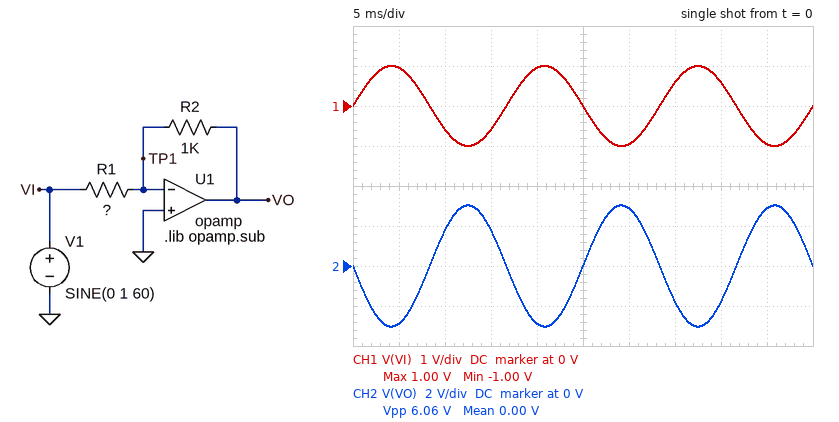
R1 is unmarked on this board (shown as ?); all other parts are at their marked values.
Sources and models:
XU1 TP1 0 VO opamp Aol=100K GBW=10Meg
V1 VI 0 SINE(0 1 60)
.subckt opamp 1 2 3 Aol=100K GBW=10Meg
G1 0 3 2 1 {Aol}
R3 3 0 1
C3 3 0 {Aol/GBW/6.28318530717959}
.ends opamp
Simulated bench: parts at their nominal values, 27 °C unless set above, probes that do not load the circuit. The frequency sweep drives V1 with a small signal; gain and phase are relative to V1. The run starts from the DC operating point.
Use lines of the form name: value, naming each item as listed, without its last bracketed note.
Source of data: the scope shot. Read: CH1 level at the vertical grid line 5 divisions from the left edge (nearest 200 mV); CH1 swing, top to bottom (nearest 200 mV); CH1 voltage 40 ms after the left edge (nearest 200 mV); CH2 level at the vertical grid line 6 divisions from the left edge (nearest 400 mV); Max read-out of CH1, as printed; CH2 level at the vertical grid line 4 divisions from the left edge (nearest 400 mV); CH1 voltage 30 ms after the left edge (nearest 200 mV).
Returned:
CH1 level at the vertical grid line 5 divisions from the left edge: 0 V
CH1 swing, top to bottom: 2.0 V
CH1 voltage 40 ms after the left edge: 600 mV
CH2 level at the vertical grid line 6 divisions from the left edge: 2.8 V
Max read-out of CH1, as printed: 1.00 V
CH2 level at the vertical grid line 4 divisions from the left edge: -2.8 V
CH1 voltage 30 ms after the left edge: -1.0 V
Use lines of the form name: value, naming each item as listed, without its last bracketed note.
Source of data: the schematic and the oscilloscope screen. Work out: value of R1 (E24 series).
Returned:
value of R1: 330 Ω
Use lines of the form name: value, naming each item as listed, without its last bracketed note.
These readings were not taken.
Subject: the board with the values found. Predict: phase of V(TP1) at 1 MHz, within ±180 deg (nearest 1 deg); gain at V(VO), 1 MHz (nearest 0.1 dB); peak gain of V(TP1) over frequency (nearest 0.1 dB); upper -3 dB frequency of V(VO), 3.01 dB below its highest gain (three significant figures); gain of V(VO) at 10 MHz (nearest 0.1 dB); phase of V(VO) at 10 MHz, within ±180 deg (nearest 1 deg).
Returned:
phase of V(TP1) at 1 MHz, within ±180 deg: 68 deg
gain at V(VO), 1 MHz: 9.0 dB
peak gain of V(TP1) over frequency: -2.5 dB
upper -3 dB frequency of V(VO), 3.01 dB below its highest gain: 2.48 MHz
gain of V(VO) at 10 MHz: -2.7 dB
phase of V(VO) at 10 MHz, within ±180 deg: 104 deg
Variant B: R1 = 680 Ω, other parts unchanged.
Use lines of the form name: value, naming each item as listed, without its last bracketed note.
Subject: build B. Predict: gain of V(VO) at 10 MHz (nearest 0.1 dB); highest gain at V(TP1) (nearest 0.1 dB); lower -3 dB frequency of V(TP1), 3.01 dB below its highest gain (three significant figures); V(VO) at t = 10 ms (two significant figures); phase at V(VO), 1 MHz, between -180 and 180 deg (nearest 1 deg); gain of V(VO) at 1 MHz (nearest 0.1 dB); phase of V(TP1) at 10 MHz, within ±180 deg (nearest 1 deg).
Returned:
gain of V(VO) at 10 MHz: -5.2 dB
highest gain at V(TP1): -4.5 dB
lower -3 dB frequency of V(TP1), 3.01 dB below its highest gain: 4.05 MHz
V(VO) at t = 10 ms: 860 mV
phase at V(VO), 1 MHz, between -180 and 180 deg: 166 deg
gain of V(VO) at 1 MHz: 3.1 dB
phase of V(TP1) at 10 MHz, within ±180 deg: 22 deg
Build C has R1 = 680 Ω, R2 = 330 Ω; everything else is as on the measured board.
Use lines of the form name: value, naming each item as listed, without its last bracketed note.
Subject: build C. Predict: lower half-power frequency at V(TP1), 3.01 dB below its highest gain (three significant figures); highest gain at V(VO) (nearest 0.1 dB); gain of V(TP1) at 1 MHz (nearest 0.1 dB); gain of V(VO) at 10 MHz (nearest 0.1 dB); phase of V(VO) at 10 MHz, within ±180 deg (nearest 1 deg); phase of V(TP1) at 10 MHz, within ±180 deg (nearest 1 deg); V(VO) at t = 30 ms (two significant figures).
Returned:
lower half-power frequency at V(TP1), 3.01 dB below its highest gain: 6.73 MHz
highest gain at V(VO): -6.3 dB
gain of V(TP1) at 1 MHz: -26.4 dB
gain of V(VO) at 10 MHz: -11.3 dB
phase of V(VO) at 10 MHz, within ±180 deg: 124 deg
phase of V(TP1) at 10 MHz, within ±180 deg: 34 deg
V(VO) at t = 30 ms: 460 mV
